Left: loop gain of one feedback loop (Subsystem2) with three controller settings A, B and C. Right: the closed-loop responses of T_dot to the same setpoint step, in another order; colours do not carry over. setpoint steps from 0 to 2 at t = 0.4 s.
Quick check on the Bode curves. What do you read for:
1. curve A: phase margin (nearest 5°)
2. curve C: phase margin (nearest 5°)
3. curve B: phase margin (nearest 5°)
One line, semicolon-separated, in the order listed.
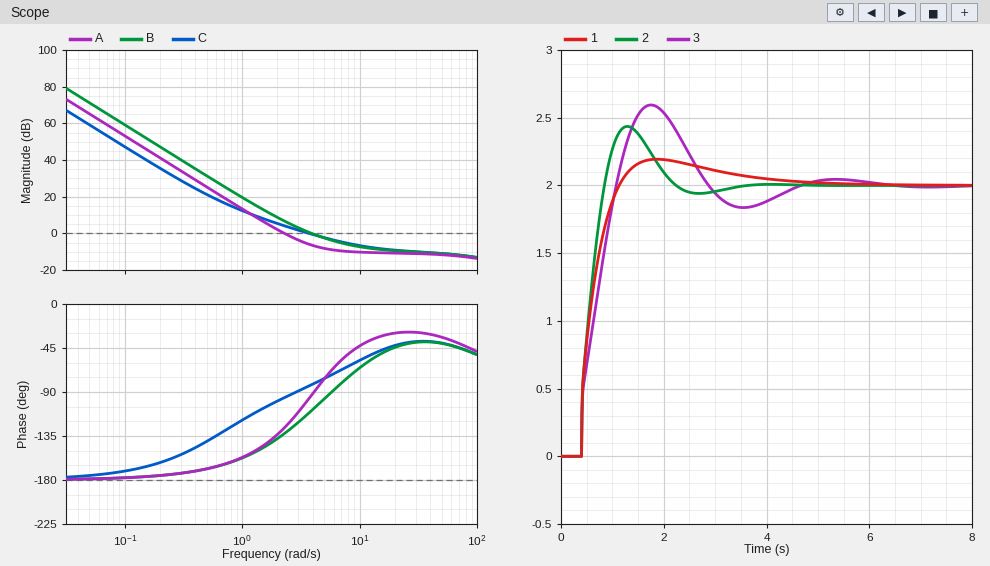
55°; 95°; 70°
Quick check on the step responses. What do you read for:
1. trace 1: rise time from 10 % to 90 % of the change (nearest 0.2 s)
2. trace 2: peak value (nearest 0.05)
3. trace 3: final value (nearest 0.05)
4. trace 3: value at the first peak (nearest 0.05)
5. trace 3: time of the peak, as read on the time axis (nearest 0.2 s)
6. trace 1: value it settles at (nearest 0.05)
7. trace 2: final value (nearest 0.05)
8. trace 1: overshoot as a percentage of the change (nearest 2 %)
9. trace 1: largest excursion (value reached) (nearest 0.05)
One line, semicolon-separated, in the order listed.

0.6 s; 2.45; 2.00; 2.60; 1.8 s; 2.00; 2.00; 10 %; 2.20
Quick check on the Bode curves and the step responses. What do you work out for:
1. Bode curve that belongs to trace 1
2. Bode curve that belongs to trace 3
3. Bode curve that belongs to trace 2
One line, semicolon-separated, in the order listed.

C; A; B
